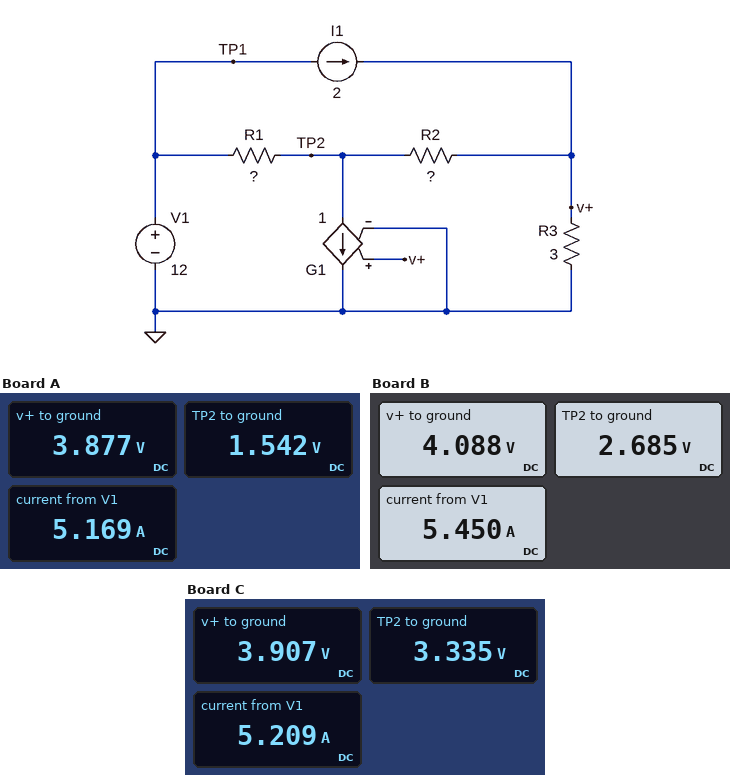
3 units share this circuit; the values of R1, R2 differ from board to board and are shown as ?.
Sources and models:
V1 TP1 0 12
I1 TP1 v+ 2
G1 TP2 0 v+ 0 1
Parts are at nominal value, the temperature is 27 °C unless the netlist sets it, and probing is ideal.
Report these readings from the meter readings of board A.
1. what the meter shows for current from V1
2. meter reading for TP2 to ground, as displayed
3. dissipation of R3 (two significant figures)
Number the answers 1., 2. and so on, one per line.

1. 5.169 A
2. 1.542 V
3. 5.0 W
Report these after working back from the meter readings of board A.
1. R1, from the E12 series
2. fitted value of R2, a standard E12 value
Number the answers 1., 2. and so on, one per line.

1. 3.3 Ω
2. 3.3 Ω
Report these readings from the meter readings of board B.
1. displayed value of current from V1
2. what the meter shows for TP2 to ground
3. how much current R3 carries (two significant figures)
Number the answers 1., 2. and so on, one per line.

1. 5.450 A
2. 2.685 V
3. 1.4 A
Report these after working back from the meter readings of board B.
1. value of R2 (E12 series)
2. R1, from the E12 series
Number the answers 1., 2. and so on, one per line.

1. 2.2 Ω
2. 2.7 Ω
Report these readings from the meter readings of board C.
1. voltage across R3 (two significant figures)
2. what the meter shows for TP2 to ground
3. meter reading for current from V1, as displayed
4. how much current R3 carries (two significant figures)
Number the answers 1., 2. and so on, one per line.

1. 3.9 V
2. 3.335 V
3. 5.209 A
4. 1.3 A
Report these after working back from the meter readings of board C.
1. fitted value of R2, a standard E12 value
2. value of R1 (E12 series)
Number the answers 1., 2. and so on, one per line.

1. 0.82 Ω
2. 2.7 Ω
